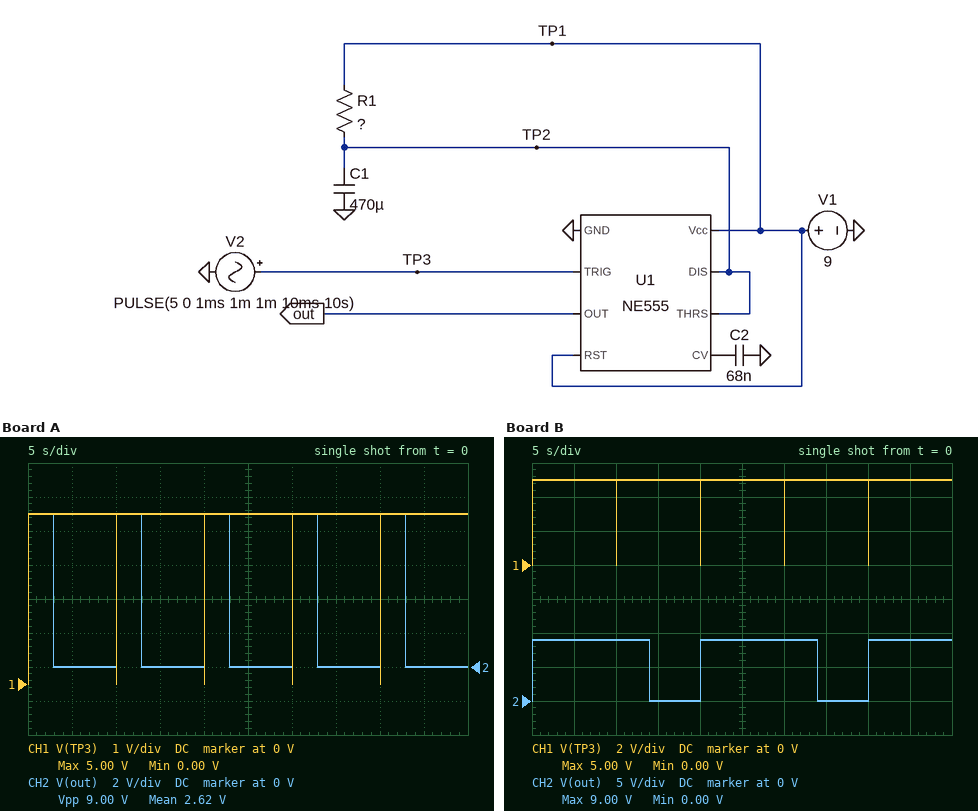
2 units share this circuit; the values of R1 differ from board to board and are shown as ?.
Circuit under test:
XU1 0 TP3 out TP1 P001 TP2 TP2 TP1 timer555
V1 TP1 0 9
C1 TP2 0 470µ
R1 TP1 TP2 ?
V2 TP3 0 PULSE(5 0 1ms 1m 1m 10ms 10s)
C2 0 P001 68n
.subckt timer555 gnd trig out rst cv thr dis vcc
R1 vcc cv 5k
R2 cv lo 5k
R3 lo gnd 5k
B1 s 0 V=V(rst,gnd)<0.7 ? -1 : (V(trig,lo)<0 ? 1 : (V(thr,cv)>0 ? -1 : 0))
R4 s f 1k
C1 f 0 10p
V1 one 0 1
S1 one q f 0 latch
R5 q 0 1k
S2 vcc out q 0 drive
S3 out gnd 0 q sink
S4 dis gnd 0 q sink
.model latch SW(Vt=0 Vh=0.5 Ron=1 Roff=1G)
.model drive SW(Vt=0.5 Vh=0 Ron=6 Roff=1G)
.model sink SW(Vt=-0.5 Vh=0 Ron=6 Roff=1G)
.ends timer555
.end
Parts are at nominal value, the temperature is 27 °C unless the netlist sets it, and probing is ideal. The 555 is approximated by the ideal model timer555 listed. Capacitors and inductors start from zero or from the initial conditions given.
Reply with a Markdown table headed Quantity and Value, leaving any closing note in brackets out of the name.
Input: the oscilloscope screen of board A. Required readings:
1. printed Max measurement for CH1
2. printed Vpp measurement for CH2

| Quantity | Value |
|---|---|
| printed Max measurement for CH1 | 5.00 V |
| printed Vpp measurement for CH2 | 9.00 V |
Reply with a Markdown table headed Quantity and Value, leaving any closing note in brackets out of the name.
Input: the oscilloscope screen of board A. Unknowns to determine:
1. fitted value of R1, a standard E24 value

| Quantity | Value |
|---|---|
| fitted value of R1, a standard E24 value | 5.6 kΩ |
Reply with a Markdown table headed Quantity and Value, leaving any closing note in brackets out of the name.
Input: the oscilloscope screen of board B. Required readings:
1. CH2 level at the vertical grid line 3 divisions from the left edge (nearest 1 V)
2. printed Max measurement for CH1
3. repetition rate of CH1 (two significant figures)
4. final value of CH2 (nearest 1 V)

| Quantity | Value |
|---|---|
| CH2 level at the vertical grid line 3 divisions from the left edge | 0 V |
| printed Max measurement for CH1 | 5.00 V |
| repetition rate of CH1 | 100 mHz |
| final value of CH2 | 9 V |
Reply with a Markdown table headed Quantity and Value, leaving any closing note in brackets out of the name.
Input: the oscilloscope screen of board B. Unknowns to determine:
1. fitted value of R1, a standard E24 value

| Quantity | Value |
|---|---|
| fitted value of R1, a standard E24 value | 27 kΩ |
